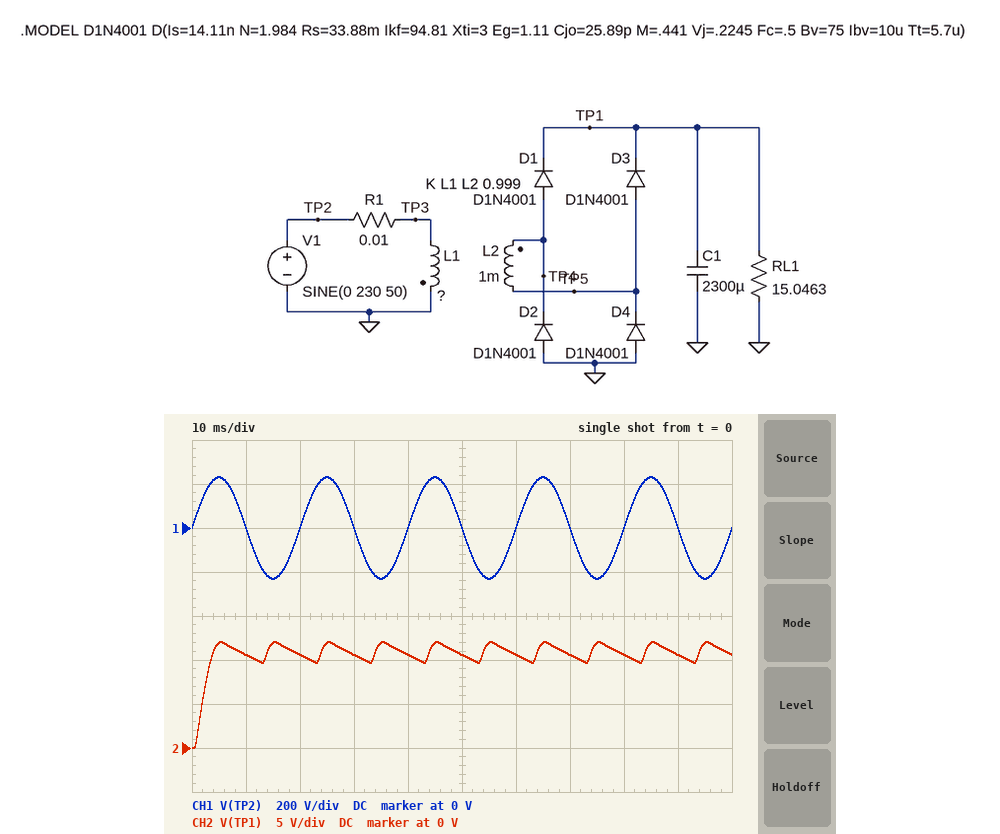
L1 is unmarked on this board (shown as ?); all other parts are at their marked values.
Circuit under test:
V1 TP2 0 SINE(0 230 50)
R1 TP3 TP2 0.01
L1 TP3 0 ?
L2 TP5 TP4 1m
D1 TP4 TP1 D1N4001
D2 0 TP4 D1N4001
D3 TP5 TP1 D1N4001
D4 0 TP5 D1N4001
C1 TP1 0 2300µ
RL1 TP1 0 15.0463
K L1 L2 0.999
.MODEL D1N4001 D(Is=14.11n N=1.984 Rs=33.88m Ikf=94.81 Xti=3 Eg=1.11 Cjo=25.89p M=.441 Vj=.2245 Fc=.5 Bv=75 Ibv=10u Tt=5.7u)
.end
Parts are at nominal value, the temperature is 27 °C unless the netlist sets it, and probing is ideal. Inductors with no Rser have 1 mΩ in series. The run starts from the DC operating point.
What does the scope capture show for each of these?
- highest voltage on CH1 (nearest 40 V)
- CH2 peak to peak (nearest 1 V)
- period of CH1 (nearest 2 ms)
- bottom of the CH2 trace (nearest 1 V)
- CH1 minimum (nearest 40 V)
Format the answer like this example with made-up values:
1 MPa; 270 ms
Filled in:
240 V; 12 V; 20 ms; 0 V; -240 V
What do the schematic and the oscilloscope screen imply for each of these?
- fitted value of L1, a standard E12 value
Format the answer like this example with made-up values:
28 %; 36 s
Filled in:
270 mH
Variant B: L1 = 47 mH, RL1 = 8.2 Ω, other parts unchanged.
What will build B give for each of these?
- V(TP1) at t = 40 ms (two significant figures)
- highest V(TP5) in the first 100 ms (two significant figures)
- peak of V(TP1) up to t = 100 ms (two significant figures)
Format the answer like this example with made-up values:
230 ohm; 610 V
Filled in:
25 V; 32 V; 31 V
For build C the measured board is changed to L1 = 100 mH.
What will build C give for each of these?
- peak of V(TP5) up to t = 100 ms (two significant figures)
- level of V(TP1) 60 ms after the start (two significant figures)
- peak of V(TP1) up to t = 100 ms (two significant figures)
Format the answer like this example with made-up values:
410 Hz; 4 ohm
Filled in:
22 V; 18 V; 21 V
